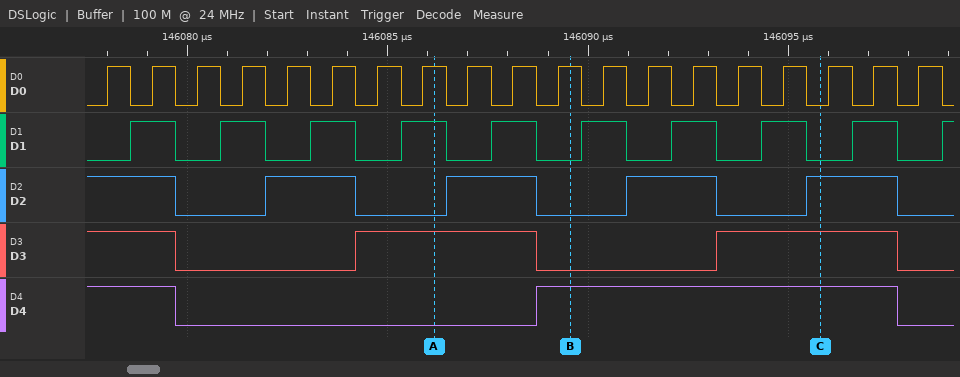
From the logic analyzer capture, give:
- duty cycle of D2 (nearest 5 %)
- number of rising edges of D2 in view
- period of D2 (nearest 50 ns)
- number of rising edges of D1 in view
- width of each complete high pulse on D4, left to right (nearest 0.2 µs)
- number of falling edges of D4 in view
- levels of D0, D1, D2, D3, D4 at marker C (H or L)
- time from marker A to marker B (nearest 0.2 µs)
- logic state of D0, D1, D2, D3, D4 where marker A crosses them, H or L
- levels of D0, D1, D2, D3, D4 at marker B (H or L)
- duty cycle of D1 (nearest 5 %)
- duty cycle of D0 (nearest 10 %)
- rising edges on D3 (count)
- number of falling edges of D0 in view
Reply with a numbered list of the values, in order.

1. 50 %
2. 4
3. 4500 ns
4. 10
5. 9 µs
6. 2
7. D0=L, D1=L, D2=H, D3=H, D4=H
8. 3.4 µs
9. D0=H, D1=H, D2=L, D3=H, D4=L
10. D0=H, D1=L, D2=L, D3=L, D4=H
11. 50 %
12. 50 %
13. 2
14. 19
